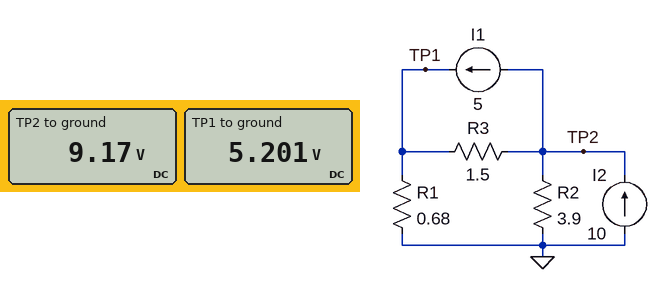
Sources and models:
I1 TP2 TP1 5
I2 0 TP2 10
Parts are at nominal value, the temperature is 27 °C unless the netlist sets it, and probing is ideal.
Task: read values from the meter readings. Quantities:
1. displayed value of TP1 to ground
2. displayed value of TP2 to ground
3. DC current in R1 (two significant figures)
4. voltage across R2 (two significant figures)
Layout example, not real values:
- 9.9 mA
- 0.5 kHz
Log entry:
- 5.201 V
- 9.17 V
- 7.6 A
- 9.2 V
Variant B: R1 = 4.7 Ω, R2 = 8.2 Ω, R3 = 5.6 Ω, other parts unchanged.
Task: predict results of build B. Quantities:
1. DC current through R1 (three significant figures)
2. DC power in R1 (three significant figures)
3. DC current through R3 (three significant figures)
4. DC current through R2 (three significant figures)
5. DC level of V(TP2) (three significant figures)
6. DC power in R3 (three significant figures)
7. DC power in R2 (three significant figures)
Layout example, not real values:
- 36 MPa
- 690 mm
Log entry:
- 5.95 A
- 166 W
- 946 mA
- 4.05 A
- 33.2 V
- 5.01 W
- 135 W
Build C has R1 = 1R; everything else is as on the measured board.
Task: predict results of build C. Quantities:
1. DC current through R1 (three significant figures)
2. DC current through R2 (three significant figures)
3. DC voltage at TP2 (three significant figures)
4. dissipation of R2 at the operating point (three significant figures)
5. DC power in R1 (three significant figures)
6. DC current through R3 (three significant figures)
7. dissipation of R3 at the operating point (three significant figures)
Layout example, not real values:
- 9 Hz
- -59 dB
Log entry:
- 7.27 A
- 2.73 A
- 10.7 V
- 29.2 W
- 52.8 W
- 2.27 A
- 7.70 W
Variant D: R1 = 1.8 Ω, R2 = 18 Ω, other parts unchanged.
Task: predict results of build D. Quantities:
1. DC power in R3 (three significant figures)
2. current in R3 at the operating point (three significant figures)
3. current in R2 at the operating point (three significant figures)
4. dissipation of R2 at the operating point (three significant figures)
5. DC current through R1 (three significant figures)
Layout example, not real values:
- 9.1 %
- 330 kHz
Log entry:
- 21.7 W
- 3.80 A
- 1.20 A
- 25.8 W
- 8.80 A
